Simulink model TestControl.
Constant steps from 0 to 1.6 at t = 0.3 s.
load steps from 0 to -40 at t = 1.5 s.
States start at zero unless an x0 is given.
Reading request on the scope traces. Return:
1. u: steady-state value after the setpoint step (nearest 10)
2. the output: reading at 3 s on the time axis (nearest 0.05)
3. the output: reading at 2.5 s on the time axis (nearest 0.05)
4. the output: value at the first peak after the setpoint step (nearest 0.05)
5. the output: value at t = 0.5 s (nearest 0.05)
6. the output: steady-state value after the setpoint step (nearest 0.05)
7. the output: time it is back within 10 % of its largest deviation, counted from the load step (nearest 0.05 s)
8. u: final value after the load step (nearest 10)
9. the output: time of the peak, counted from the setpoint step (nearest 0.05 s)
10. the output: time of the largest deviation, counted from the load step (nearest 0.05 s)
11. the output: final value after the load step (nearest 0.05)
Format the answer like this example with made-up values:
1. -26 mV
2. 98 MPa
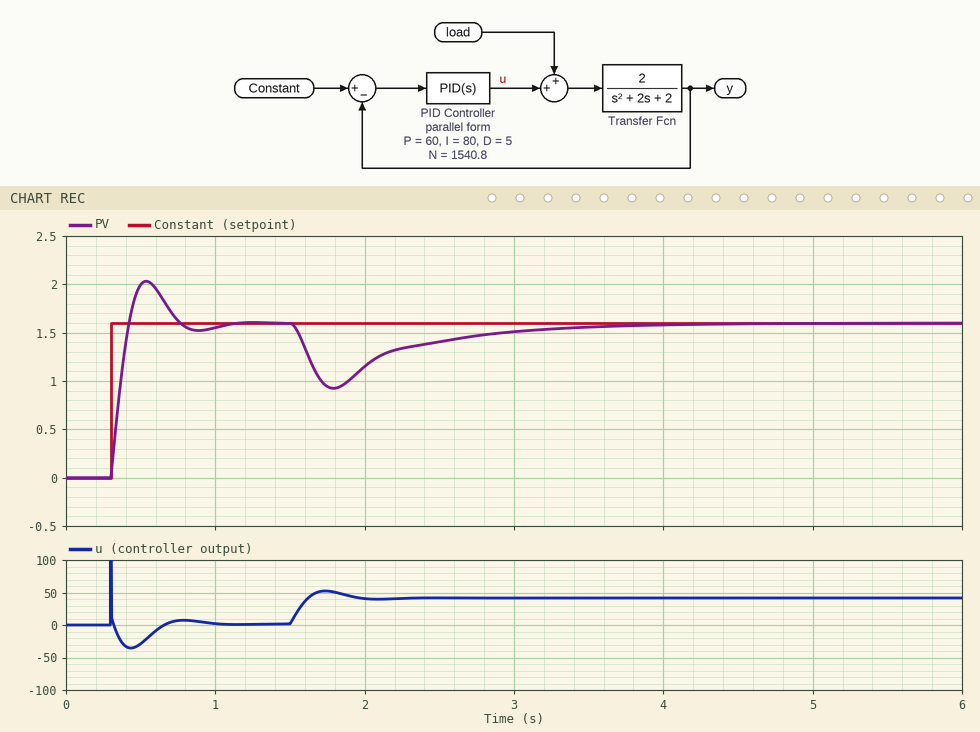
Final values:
1. 0
2. 1.50
3. 1.40
4. 2.05
5. 2.00
6. 1.60
7. 1.70 s
8. 40
9. 0.25 s
10. 0.30 s
11. 1.60
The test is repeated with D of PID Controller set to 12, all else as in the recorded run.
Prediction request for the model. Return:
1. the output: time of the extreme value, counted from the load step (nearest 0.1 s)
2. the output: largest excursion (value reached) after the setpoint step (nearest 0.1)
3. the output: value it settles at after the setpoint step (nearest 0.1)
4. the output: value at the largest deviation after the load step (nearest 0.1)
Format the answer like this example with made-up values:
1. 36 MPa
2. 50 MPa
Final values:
1. 0.4 s
2. 1.7
3. 1.6
4. 1.1
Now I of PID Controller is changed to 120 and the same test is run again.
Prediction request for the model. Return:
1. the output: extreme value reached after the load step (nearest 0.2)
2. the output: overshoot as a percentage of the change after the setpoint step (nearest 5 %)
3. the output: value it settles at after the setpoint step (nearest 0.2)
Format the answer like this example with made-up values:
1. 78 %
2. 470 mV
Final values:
1. 1.0
2. 30 %
3. 1.6
